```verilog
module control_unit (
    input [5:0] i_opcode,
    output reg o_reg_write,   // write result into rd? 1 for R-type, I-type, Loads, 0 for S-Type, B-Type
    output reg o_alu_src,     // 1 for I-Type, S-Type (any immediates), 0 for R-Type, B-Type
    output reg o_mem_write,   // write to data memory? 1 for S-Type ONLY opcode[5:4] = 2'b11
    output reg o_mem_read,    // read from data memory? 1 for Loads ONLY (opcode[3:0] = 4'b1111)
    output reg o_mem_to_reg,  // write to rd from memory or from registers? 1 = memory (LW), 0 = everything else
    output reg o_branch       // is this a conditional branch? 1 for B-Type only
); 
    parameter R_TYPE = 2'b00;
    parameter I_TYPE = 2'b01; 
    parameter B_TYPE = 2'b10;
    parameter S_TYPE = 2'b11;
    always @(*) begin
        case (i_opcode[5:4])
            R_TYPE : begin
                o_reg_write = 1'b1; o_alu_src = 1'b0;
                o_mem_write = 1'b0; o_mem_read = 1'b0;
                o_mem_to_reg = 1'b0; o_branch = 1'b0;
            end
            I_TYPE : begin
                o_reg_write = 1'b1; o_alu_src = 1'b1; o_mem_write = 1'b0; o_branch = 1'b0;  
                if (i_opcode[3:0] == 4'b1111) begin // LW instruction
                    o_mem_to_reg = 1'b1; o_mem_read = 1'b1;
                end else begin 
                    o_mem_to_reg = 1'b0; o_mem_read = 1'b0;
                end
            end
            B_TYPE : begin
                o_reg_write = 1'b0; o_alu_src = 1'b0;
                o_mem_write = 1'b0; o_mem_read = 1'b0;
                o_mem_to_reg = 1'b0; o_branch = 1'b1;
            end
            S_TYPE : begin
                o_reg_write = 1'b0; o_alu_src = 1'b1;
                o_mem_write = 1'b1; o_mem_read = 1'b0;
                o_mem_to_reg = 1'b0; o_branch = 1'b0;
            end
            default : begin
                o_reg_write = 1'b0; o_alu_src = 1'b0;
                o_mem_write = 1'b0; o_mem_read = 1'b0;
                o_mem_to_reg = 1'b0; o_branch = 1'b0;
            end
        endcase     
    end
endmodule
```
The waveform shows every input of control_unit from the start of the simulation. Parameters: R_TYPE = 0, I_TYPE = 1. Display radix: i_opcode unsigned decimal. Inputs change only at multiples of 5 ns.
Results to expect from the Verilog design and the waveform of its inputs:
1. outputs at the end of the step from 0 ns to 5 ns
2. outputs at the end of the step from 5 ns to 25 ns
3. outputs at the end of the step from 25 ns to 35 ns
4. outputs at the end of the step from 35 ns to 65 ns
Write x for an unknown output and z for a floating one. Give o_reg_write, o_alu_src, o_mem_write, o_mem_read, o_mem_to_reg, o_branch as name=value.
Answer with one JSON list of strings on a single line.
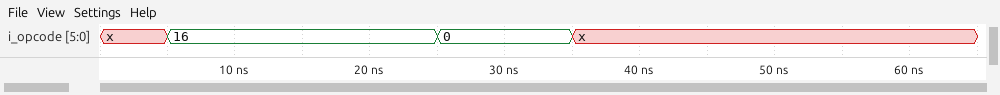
["o_reg_write=x, o_alu_src=x, o_mem_write=x, o_mem_read=x, o_mem_to_reg=x, o_branch=x", "o_reg_write=1, o_alu_src=1, o_mem_write=0, o_mem_read=0, o_mem_to_reg=0, o_branch=0", "o_reg_write=1, o_alu_src=0, o_mem_write=0, o_mem_read=0, o_mem_to_reg=0, o_branch=0", "o_reg_write=0, o_alu_src=0, o_mem_write=0, o_mem_read=0, o_mem_to_reg=0, o_branch=0"]
